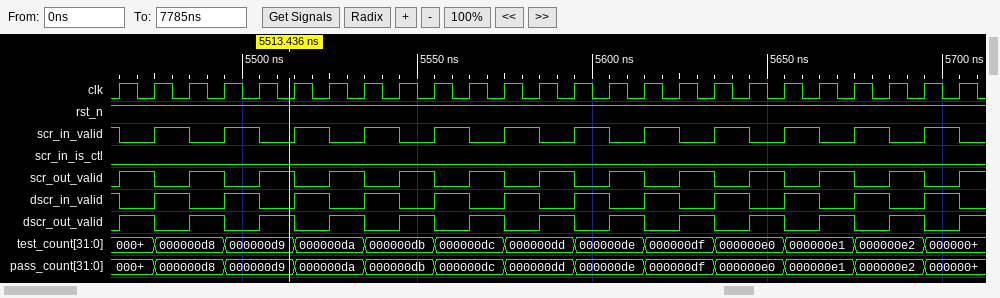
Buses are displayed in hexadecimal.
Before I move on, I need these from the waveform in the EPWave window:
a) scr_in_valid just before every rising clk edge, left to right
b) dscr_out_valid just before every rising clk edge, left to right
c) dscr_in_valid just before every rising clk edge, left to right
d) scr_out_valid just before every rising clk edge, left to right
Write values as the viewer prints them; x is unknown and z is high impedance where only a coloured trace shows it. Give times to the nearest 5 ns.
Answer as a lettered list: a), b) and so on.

a) 1 0 1 0 1 0 1 0 1 0 1 0 1 0 1 0 1 0 1 0 1 0 1 0 1
b) 0 1 0 1 0 1 0 1 0 1 0 1 0 1 0 1 0 1 0 1 0 1 0 1 0
c) 1 0 1 0 1 0 1 0 1 0 1 0 1 0 1 0 1 0 1 0 1 0 1 0 1
d) 0 1 0 1 0 1 0 1 0 1 0 1 0 1 0 1 0 1 0 1 0 1 0 1 0
